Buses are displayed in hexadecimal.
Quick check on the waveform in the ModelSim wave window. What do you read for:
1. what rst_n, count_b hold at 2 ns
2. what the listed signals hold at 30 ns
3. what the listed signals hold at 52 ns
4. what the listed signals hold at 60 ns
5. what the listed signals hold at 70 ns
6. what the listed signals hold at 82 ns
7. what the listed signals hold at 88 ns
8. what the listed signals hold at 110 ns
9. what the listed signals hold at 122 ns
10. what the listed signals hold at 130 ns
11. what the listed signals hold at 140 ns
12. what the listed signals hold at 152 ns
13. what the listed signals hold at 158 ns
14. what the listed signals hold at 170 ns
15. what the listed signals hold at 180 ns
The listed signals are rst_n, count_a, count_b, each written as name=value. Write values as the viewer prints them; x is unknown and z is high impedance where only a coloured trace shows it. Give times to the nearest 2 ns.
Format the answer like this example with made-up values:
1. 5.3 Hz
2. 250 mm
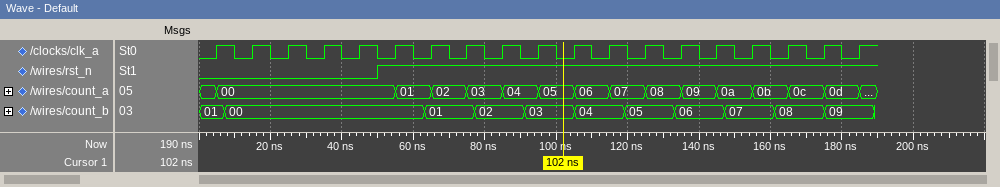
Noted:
1. rst_n=0, count_b=01
2. rst_n=0, count_a=00, count_b=00
3. rst_n=1, count_a=00, count_b=00
4. rst_n=1, count_a=01, count_b=00
5. rst_n=1, count_a=02, count_b=01
6. rst_n=1, count_a=03, count_b=02
7. rst_n=1, count_a=04, count_b=02
8. rst_n=1, count_a=06, count_b=04
9. rst_n=1, count_a=07, count_b=05
10. rst_n=1, count_a=08, count_b=05
11. rst_n=1, count_a=09, count_b=06
12. rst_n=1, count_a=0a, count_b=07
13. rst_n=1, count_a=0b, count_b=07
14. rst_n=1, count_a=0c, count_b=08
15. rst_n=1, count_a=0d, count_b=09
